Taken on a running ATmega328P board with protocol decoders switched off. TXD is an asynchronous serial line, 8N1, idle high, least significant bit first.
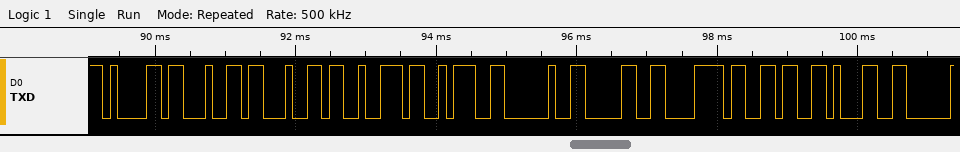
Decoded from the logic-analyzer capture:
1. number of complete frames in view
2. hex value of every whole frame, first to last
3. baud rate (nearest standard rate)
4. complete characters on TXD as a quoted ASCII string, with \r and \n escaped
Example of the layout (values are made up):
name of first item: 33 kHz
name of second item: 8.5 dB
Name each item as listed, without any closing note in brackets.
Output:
number of complete frames in view: 10
hex value of every whole frame, first to last: 61 64 64 72 3A 20 30 78 36 31
baud rate: 9600 baud
complete characters on TXD as a quoted ASCII string, with \r and \n escaped: "addr: 0x61"
